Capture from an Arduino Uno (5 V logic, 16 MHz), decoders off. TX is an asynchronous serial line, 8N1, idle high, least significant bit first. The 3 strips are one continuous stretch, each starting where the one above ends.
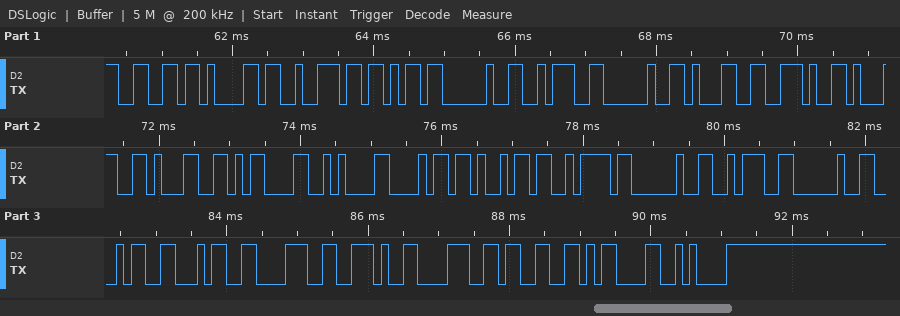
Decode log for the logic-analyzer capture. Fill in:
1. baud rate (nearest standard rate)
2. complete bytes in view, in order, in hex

9600 baud
66 61 72 6B 20 3A 20 31 2E 31 31 0D 0A 68 69 7A 20 3A 20 34 34 38 2E 38 33 0D 0A
